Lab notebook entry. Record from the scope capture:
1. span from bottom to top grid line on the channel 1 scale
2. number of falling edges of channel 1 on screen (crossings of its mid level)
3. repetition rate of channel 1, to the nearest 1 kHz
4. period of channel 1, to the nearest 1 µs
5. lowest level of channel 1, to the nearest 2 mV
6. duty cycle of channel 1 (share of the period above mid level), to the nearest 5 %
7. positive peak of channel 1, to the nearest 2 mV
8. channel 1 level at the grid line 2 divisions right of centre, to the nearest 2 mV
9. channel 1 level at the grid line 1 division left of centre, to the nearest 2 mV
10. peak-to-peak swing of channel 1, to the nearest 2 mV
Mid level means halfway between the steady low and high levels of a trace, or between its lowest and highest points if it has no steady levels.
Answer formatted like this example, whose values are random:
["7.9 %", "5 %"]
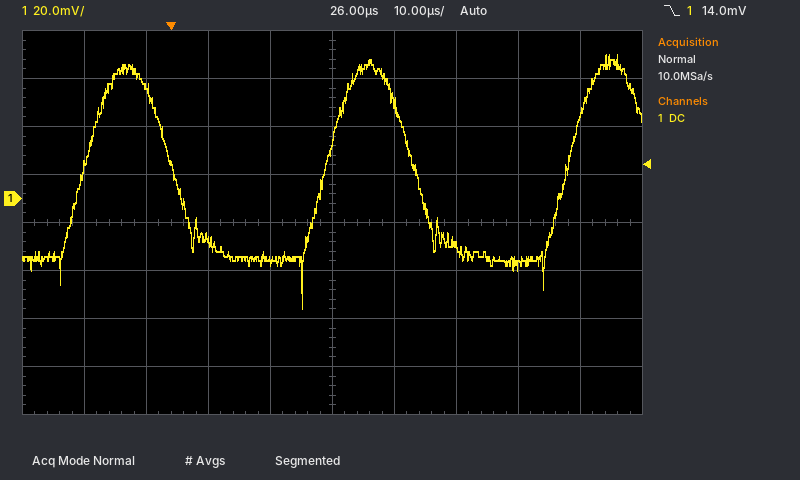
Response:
["160 mV", "2", "26 kHz", "39 µs", "-46 mV", "40 %", "60 mV", "-20 mV", "-26 mV", "106 mV"]
